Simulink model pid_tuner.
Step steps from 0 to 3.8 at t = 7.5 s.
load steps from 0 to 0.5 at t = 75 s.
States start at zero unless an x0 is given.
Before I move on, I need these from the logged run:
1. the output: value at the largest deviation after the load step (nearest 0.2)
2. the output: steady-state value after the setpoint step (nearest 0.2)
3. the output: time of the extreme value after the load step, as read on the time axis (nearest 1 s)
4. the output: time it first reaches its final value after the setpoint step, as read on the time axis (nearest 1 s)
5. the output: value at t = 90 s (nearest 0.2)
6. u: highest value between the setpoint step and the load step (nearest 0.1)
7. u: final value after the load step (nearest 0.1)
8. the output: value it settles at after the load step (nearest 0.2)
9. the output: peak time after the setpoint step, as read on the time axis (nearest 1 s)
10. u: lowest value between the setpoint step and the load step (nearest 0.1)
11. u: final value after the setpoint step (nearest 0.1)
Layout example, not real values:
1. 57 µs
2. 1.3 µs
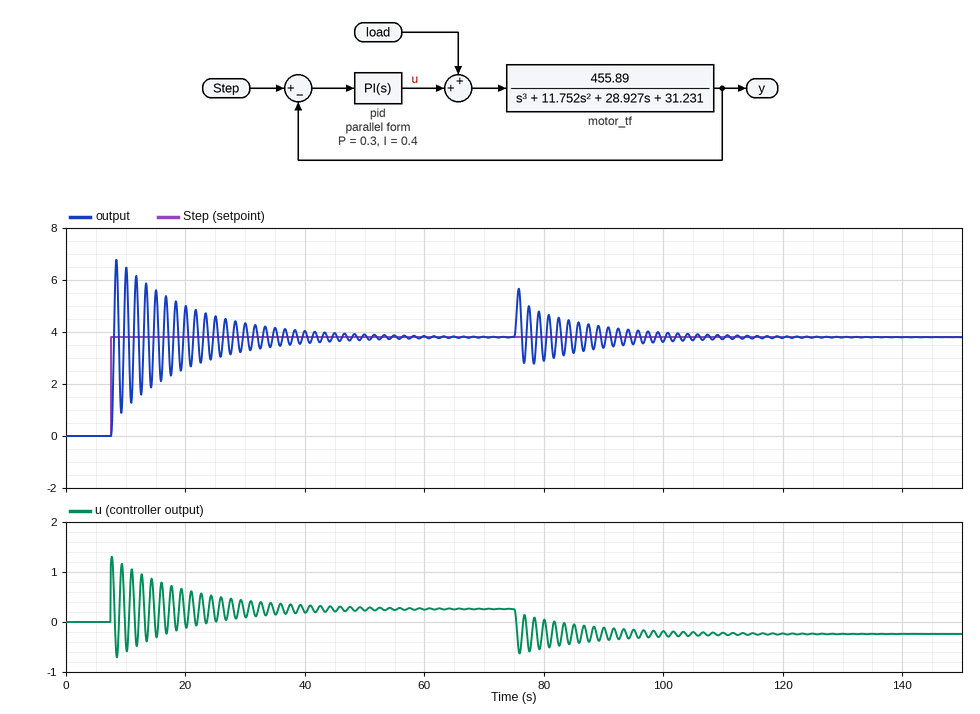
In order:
1. 5.6
2. 3.8
3. 76 s
4. 8 s
5. 3.4
6. 1.3
7. -0.2
8. 3.8
9. 8 s
10. -0.7
11. 0.3
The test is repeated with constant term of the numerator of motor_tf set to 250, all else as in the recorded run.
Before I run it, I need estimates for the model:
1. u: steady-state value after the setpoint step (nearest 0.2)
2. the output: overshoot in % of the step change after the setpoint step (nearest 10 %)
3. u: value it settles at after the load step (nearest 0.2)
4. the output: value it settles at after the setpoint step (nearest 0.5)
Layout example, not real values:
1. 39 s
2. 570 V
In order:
1. 0.4
2. 50 %
3. 0.0
4. 4.0
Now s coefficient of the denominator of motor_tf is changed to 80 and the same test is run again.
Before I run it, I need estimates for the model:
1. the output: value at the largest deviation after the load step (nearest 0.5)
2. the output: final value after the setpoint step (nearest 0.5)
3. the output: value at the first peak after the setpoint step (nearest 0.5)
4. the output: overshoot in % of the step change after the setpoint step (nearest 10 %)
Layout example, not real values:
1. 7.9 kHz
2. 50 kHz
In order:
1. 5.0
2. 4.0
3. 4.5
4. 20 %
